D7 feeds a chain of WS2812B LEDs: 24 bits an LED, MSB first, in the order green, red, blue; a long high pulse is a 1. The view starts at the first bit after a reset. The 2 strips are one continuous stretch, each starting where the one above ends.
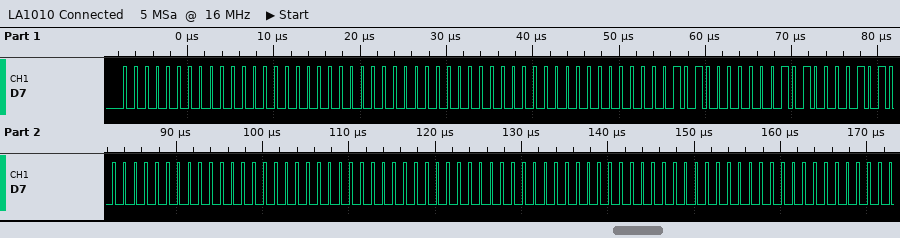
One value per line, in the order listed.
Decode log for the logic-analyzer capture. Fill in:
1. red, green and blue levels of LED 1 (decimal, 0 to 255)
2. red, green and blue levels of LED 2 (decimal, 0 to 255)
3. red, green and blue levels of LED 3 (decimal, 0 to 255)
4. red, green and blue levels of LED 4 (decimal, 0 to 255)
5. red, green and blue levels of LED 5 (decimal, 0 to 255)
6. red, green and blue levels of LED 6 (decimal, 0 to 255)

0, 0, 0
0, 0, 0
5, 20, 10
0, 0, 0
0, 0, 0
0, 0, 0
